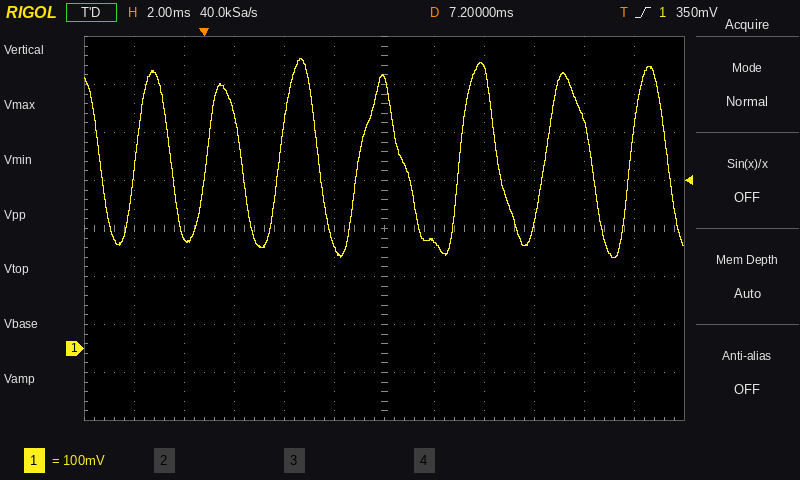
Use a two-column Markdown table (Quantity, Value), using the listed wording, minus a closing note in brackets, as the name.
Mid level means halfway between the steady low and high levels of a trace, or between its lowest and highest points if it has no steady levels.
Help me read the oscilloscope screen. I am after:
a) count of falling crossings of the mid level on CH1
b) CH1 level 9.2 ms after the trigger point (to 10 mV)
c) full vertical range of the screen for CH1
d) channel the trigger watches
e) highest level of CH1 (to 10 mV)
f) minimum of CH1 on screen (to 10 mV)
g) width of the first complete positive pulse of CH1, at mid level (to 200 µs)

| Quantity | Value |
|---|---|
| count of falling crossings of the mid level on CH1 | 8 |
| CH1 level 9.2 ms after the trigger point | 220 mV |
| full vertical range of the screen for CH1 | 800 mV |
| channel the trigger watches | CH1 |
| highest level of CH1 | 600 mV |
| minimum of CH1 on screen | 190 mV |
| width of the first complete positive pulse of CH1, at mid level | 1.4 ms |
